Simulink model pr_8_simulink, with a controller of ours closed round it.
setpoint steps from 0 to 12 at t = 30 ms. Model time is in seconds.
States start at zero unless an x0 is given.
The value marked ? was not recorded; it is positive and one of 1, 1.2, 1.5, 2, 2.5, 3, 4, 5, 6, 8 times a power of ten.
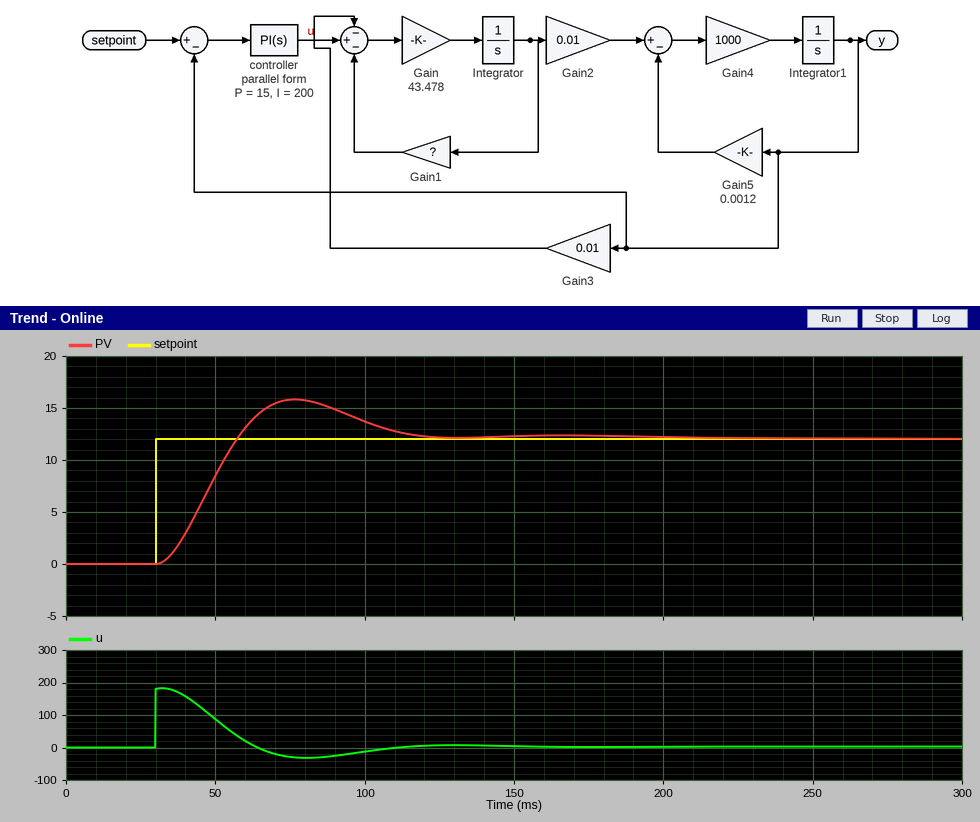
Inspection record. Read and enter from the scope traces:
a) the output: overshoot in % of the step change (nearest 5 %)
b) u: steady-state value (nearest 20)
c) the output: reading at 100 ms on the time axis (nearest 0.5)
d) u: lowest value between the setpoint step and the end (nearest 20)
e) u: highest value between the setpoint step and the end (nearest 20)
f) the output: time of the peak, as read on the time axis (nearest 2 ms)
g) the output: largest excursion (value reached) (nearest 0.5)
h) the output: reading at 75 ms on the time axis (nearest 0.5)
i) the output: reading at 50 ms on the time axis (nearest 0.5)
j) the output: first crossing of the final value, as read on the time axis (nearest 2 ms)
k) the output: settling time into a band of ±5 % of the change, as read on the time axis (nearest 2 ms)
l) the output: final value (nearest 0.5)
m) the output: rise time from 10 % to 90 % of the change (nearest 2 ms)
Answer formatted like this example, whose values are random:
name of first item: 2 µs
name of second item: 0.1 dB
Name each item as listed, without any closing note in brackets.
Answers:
the output: overshoot in % of the step change: 30 %
u: steady-state value: 0
the output: reading at 100 ms on the time axis: 13.5
u: lowest value between the setpoint step and the end: -40
u: highest value between the setpoint step and the end: 180
the output: time of the peak, as read on the time axis: 76 ms
the output: largest excursion (value reached): 16.0
the output: reading at 75 ms on the time axis: 16.0
the output: reading at 50 ms on the time axis: 8.5
the output: first crossing of the final value, as read on the time axis: 58 ms
the output: settling time into a band of ±5 % of the change, as read on the time axis: 112 ms
the output: final value: 12.0
the output: rise time from 10 % to 90 % of the change: 18 ms
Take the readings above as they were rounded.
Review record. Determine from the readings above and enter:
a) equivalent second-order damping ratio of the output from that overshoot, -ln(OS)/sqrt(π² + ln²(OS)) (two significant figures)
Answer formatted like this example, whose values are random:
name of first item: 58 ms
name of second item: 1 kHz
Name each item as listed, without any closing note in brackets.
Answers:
equivalent second-order damping ratio of the output from that overshoot, -ln(OS)/sqrt(π² + ln²(OS)): 0.36
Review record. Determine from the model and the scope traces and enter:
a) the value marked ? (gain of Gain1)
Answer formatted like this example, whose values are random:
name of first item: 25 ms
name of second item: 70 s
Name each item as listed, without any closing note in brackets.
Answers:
the value marked ?: 2
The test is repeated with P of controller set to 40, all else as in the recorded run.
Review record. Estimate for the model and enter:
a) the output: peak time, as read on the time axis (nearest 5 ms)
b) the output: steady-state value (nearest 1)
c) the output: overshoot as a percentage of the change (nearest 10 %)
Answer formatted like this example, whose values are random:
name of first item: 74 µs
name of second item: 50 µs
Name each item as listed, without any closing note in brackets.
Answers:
the output: peak time, as read on the time axis: 55 ms
the output: steady-state value: 12
the output: overshoot as a percentage of the change: 40 %
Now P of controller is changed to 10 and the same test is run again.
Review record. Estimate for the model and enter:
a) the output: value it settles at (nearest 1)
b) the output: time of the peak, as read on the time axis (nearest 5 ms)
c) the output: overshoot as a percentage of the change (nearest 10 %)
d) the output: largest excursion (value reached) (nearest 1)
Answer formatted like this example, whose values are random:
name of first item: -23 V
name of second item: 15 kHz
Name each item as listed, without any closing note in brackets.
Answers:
the output: value it settles at: 12
the output: time of the peak, as read on the time axis: 90 ms
the output: overshoot as a percentage of the change: 40 %
the output: largest excursion (value reached): 17
